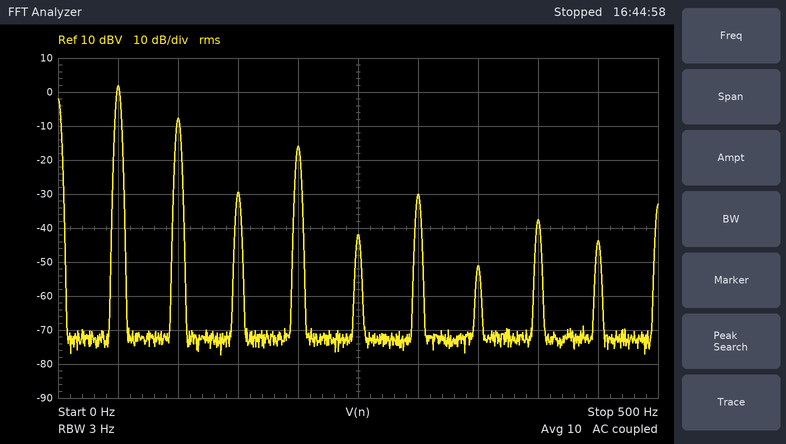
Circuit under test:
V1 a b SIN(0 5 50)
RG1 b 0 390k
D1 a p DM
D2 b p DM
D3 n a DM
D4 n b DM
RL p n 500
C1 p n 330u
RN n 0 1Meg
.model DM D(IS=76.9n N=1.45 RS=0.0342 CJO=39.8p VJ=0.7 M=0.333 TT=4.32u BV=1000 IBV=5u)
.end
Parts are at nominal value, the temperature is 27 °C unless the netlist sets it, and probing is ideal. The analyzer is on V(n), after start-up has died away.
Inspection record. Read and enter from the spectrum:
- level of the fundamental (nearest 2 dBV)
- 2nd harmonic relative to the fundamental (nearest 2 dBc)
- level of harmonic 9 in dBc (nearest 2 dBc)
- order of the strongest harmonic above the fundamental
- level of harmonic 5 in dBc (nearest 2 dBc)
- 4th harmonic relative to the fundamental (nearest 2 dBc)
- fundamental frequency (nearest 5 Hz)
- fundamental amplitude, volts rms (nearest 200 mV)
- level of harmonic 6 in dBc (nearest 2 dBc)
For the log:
2 dBV
-10 dBc
-46 dBc
2
-44 dBc
-18 dBc
50 Hz
1.2 V
-32 dBc
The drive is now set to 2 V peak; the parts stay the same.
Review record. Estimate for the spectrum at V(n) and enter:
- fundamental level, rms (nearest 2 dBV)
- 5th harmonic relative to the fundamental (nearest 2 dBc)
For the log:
-6 dBV
-32 dBc
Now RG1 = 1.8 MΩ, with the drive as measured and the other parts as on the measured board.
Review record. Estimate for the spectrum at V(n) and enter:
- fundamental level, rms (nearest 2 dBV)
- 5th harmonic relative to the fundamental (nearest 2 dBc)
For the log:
-4 dBV
-40 dBc
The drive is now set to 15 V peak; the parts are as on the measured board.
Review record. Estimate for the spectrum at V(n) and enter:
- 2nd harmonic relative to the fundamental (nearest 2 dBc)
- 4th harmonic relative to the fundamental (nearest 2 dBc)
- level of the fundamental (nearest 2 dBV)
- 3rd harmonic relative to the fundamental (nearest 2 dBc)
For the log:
-8 dBc
-20 dBc
12 dBV
-38 dBc
